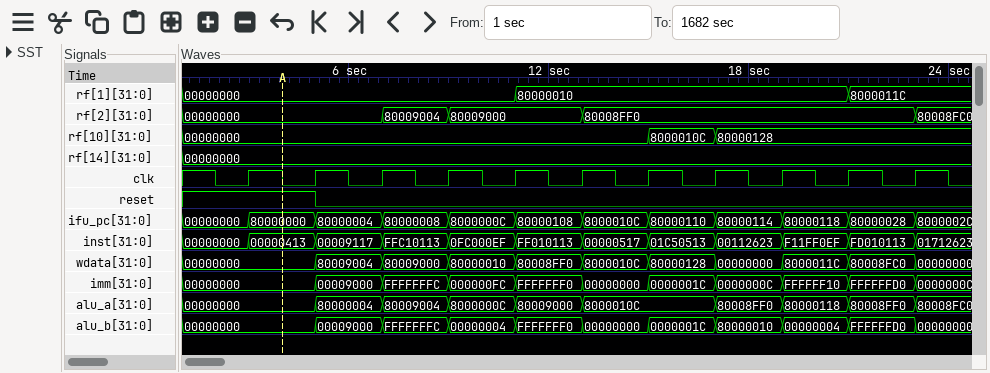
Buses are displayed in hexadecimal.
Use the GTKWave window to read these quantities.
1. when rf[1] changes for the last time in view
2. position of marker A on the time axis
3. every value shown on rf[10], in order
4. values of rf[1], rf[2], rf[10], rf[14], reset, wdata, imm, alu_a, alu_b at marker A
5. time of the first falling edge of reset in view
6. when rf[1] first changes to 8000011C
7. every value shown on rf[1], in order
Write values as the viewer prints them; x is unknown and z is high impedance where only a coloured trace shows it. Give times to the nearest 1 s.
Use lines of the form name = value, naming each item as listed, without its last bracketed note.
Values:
when rf[1] changes for the last time in view = 21 s
position of marker A on the time axis = 4 s
every value shown on rf[10], in order = 00000000, 8000010C, 80000128
values of rf[1], rf[2], rf[10], rf[14], reset, wdata, imm, alu_a, alu_b at marker A = rf[1]=00000000, rf[2]=00000000, rf[10]=00000000, rf[14]=00000000, reset=1, wdata=00000000, imm=00000000, alu_a=00000000, alu_b=00000000
time of the first falling edge of reset in view = 5 s
when rf[1] first changes to 8000011C = 21 s
every value shown on rf[1], in order = 00000000, 80000010, 8000011C
